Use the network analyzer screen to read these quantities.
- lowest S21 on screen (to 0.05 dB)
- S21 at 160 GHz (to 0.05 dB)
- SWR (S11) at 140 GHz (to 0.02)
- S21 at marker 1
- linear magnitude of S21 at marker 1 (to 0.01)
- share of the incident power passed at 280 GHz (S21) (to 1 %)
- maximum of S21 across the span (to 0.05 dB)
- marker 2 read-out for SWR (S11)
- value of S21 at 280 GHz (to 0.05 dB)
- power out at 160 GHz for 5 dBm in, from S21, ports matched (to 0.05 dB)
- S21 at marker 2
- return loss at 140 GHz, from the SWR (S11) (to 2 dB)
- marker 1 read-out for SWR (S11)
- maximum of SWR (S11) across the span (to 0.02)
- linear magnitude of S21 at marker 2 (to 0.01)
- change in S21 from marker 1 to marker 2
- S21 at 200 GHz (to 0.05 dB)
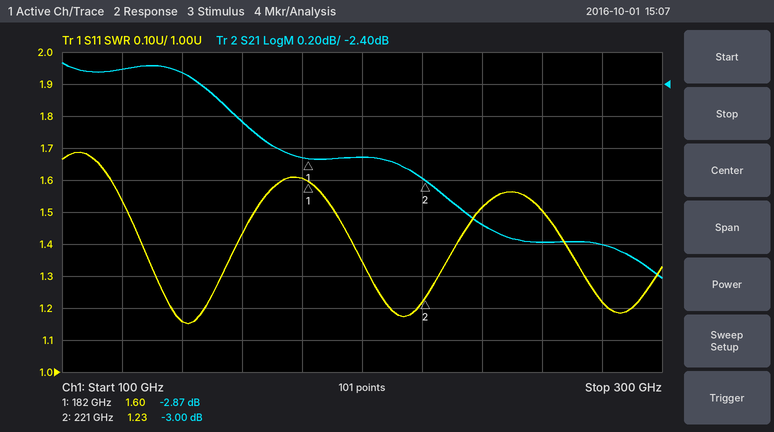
-3.60 dB
-2.65 dB
1.16
-2.87 dB
0.72
46 %
-2.25 dB
1.23
-3.40 dB
2.35 dBm
-3.00 dB
22 dB
1.60
1.68
0.71
-0.13 dB
-2.85 dB
